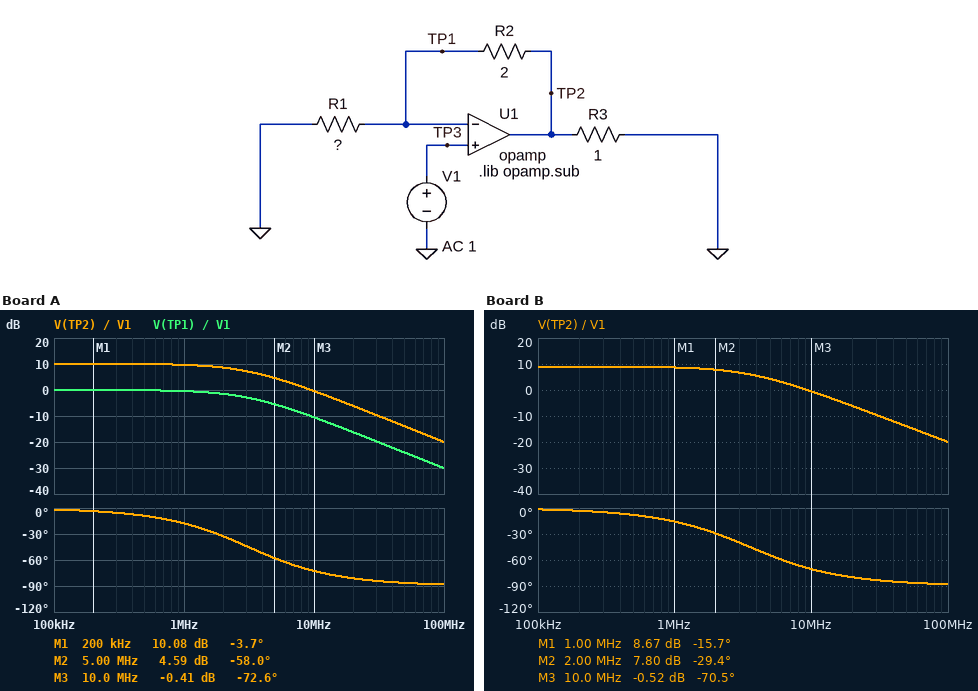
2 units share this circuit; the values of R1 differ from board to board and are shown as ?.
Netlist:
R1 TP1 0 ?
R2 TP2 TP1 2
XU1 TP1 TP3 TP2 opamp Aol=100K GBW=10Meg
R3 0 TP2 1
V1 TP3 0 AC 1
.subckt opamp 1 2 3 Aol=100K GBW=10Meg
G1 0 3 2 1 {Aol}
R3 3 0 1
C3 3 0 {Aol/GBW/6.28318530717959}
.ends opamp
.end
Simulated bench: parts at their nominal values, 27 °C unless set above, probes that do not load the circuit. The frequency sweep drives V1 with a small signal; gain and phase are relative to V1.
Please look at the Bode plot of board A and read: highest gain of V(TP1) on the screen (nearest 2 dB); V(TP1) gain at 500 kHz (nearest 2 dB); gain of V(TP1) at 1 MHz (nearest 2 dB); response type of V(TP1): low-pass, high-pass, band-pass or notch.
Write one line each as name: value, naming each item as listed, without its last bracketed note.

highest gain of V(TP1) on the screen: 0 dB
V(TP1) gain at 500 kHz: 0 dB
gain of V(TP1) at 1 MHz: 0 dB
response type of V(TP1): low-pass, high-pass, band-pass or notch: low-pass
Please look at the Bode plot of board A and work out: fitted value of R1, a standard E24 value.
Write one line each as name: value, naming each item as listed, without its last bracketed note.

fitted value of R1, a standard E24 value: 0.91 Ω
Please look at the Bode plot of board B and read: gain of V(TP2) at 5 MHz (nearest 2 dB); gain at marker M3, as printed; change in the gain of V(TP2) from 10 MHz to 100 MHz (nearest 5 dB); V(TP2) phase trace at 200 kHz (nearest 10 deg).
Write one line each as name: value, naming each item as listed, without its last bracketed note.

gain of V(TP2) at 5 MHz: 4 dB
gain at marker M3, as printed: -0.52 dB
change in the gain of V(TP2) from 10 MHz to 100 MHz: -20 dB
V(TP2) phase trace at 200 kHz: 0 deg
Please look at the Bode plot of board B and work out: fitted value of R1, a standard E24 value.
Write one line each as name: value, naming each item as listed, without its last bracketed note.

fitted value of R1, a standard E24 value: 1.1 Ω
